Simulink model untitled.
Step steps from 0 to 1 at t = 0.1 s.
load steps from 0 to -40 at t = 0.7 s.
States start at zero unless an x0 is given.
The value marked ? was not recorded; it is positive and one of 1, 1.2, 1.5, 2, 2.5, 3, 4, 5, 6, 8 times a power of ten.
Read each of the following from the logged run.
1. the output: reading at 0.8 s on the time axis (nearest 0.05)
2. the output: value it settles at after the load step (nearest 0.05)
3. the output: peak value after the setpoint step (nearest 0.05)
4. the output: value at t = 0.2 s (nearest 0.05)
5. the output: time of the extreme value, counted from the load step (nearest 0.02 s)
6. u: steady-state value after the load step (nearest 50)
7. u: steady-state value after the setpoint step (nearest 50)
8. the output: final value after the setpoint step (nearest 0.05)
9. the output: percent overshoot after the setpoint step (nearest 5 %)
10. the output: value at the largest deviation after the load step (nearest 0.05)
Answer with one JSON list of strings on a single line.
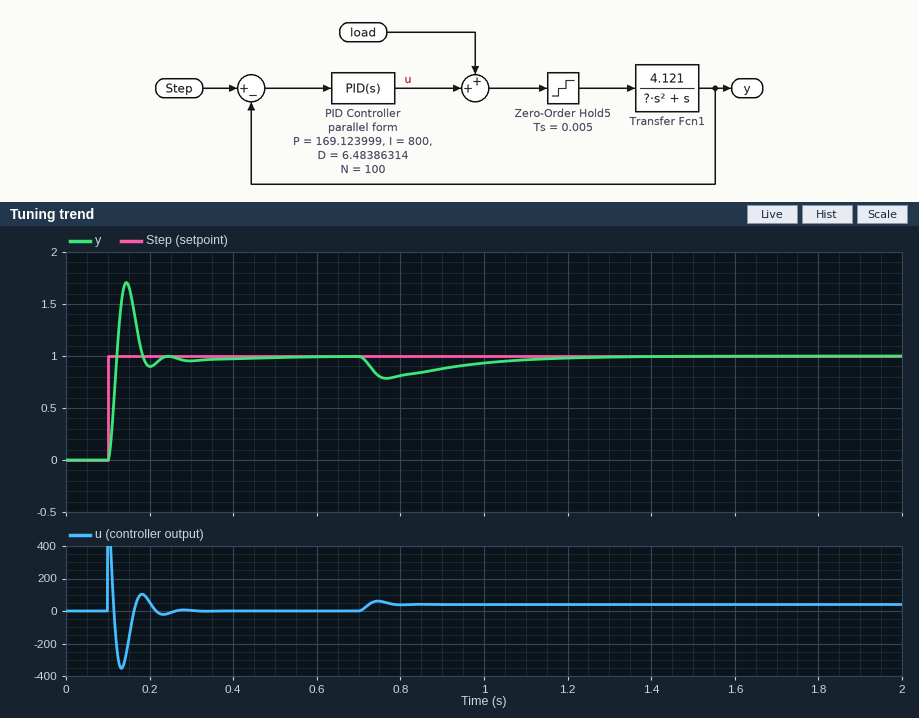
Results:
["0.80", "1.00", "1.70", "0.90", "0.06 s", "50", "0", "1.00", "70 %", "0.80"]
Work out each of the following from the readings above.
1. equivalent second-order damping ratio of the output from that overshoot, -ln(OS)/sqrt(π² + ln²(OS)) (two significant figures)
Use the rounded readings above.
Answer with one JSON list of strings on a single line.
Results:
["0.11"]
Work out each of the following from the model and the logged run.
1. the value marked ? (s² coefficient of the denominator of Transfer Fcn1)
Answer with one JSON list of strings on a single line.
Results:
["0.5"]
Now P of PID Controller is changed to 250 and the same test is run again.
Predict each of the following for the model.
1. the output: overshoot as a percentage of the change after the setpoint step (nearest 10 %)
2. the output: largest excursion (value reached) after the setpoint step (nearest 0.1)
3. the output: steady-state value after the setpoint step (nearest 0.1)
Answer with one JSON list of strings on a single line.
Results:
["80 %", "1.8", "1.0"]
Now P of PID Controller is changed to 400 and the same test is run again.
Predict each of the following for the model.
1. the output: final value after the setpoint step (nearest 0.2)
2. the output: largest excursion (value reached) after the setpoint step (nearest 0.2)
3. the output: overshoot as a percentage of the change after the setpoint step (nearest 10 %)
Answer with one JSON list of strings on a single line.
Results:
["1.0", "2.0", "90 %"]
